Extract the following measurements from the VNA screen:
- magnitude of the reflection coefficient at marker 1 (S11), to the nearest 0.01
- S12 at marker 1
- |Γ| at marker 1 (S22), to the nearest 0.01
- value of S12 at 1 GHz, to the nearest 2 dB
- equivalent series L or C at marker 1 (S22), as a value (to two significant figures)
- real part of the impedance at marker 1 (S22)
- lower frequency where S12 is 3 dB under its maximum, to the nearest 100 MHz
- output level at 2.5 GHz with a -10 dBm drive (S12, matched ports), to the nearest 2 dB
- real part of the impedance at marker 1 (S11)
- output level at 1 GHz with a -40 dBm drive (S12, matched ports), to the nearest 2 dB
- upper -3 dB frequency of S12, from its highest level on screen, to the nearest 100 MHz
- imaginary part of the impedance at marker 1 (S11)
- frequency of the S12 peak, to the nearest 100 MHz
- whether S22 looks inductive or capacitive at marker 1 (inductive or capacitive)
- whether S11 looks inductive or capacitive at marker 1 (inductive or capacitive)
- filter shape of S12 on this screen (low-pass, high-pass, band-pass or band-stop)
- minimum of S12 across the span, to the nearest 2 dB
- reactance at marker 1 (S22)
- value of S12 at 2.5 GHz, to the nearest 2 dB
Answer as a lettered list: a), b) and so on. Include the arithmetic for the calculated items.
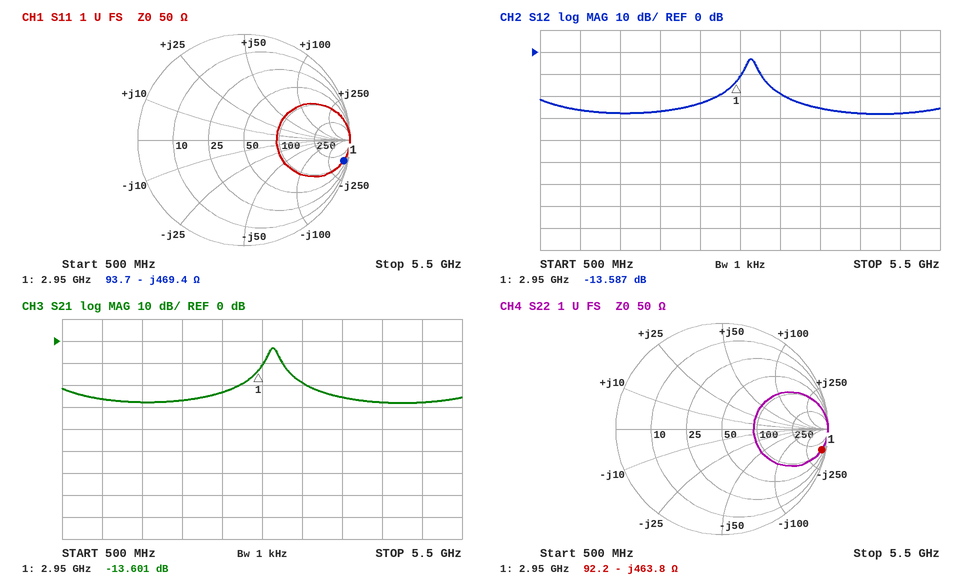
a) 0.96
b) -13.587 dB
c) 0.96
d) -26 dB
e) C = 1/(2π × 2.95 GHz × 463.8 Ω) ≈ 116 fF, so 120 fF to two significant figures
f) 92.2 Ω
g) 3.1 GHz
h) -10 dBm + (-24 dB) = -34 dBm
i) 93.7 Ω
j) -40 dBm + (-26 dB) = -66 dBm
k) 3.2 GHz
l) -469.4 Ω
m) 3.1 GHz
n) capacitive
o) capacitive
p) band-pass
q) -28 dB
r) -463.8 Ω
s) -24 dB
